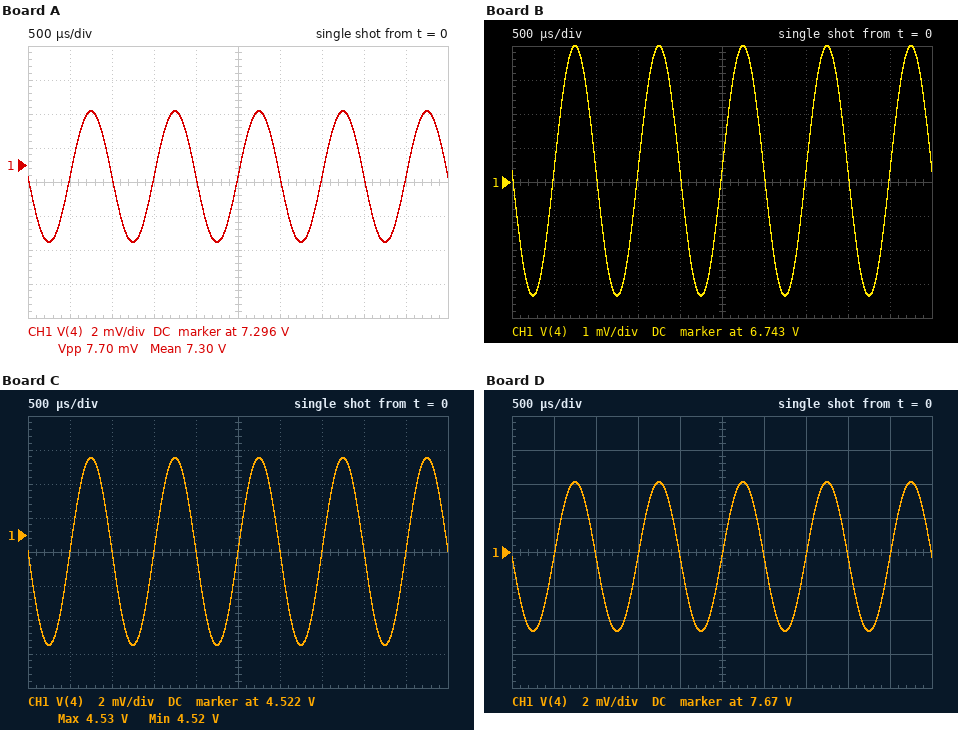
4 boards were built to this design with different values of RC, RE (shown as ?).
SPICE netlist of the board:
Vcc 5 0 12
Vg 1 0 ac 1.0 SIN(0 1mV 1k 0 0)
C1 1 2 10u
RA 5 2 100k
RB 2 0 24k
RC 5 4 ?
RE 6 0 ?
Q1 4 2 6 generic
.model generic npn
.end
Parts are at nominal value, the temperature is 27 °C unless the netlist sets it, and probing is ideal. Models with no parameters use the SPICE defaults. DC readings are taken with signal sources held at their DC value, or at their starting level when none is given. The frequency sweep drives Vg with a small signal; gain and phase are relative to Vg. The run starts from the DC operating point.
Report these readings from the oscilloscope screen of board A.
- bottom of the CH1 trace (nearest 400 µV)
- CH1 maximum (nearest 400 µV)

7.2916 V
7.2992 V
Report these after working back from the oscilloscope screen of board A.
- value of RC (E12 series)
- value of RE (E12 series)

2.7 kΩ
680 Ω
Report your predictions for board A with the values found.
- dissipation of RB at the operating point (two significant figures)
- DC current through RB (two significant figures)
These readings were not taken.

160 µW
83 µA
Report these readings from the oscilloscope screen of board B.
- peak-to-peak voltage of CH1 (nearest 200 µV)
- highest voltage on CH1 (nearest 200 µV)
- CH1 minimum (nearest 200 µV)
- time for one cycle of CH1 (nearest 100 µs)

7.4 mV
6.7470 V
6.7396 V
1.0 ms
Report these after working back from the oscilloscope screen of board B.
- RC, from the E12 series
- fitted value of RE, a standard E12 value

6.8 kΩ
1.8 kΩ
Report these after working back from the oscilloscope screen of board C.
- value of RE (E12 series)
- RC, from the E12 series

1.2 kΩ
6.8 kΩ
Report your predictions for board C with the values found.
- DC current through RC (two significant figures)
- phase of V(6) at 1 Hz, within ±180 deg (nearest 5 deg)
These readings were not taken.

1.1 mA
45 deg
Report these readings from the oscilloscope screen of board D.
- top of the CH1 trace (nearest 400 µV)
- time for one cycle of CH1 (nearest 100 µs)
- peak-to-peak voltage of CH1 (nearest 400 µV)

7.6740 V
1.0 ms
8.8 mV
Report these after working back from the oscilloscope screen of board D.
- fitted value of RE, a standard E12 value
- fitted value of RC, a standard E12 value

330 Ω
1.5 kΩ
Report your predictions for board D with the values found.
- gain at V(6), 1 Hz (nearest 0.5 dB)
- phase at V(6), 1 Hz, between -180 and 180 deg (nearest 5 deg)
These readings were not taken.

-4.5 dB
50 deg
